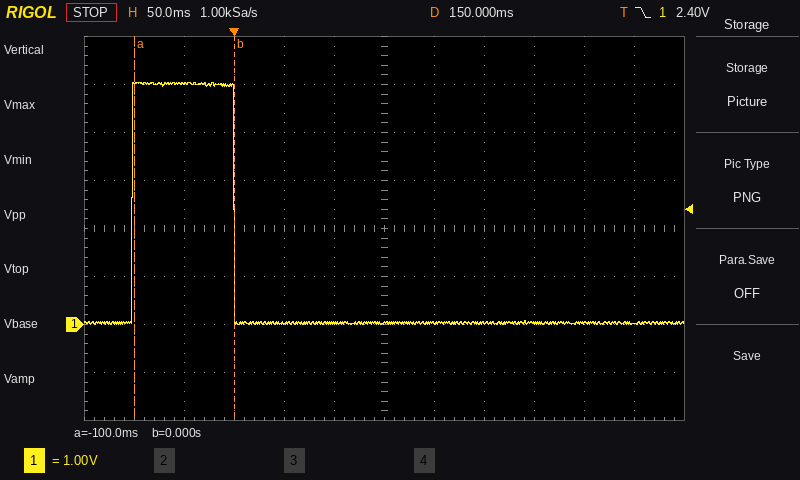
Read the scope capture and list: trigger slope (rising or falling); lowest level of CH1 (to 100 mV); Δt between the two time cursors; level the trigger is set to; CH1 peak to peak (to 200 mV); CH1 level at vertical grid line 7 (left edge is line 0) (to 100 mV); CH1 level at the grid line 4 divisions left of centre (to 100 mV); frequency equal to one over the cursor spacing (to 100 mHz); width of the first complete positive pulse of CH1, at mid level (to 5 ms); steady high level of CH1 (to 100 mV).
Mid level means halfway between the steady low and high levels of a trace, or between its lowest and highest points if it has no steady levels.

falling
0.0 V
100 ms
2.40 V
5.0 V
0.0 V
5.0 V
10.0 Hz
100 ms
5.0 V
